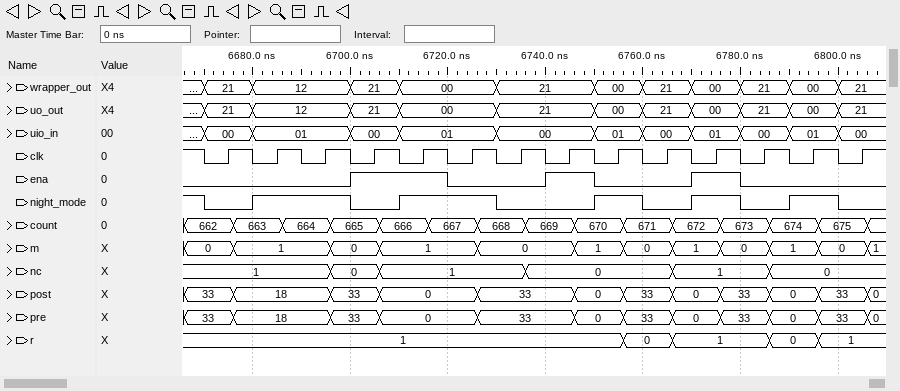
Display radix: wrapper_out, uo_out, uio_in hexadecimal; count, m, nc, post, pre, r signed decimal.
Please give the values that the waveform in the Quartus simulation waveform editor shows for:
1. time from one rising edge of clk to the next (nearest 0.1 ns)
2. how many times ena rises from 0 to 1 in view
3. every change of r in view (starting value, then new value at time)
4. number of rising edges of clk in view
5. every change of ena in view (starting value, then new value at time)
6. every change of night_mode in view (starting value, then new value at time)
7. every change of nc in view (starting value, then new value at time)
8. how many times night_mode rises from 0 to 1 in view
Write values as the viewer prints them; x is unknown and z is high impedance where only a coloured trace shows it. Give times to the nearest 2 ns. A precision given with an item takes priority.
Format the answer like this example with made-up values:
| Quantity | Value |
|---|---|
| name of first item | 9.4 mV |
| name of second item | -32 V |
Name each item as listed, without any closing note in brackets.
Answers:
| Quantity | Value |
|---|---|
| time from one rising edge of clk to the next | 10 ns |
| how many times ena rises from 0 to 1 in view | 3 |
| every change of r in view | 1, 0 at 6756 ns, 1 at 6766 ns, 0 at 6786 ns, 1 at 6796 ns |
| number of rising edges of clk in view | 14 |
| every change of ena in view | 0, 1 at 6700 ns, 0 at 6720 ns, 1 at 6740 ns, 0 at 6750 ns, 1 at 6770 ns, 0 at 6780 ns |
| every change of night_mode in view | 1, 0 at 6670 ns, 1 at 6680 ns, 0 at 6700 ns, 1 at 6710 ns, 0 at 6730 ns, 1 at 6750 ns, 0 at 6760 ns, 1 at 6770 ns, 0 at 6780 ns, 1 at 6790 ns, 0 at 6800 ns |
| every change of nc in view | 1, 0 at 6696 ns, 1 at 6706 ns, 0 at 6736 ns, 1 at 6766 ns, 0 at 6786 ns |
| how many times night_mode rises from 0 to 1 in view | 5 |
